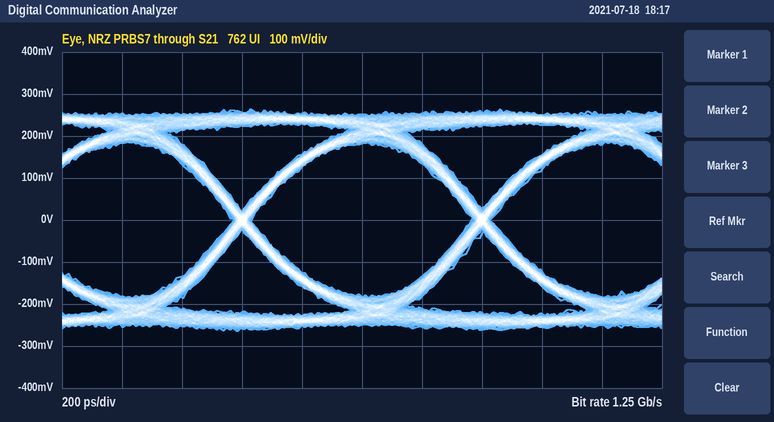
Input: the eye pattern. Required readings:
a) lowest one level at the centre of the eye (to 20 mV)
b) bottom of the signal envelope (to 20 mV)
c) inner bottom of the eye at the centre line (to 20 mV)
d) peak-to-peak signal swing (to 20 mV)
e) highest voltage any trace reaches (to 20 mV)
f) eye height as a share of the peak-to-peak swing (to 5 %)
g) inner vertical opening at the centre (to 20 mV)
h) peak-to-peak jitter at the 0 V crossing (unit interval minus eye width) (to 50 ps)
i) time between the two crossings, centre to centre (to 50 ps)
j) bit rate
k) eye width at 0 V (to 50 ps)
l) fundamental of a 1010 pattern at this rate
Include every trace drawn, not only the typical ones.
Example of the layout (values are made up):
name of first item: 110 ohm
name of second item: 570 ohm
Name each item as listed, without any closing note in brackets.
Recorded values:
lowest one level at the centre of the eye: 180 mV
bottom of the signal envelope: -260 mV
inner bottom of the eye at the centre line: -180 mV
peak-to-peak signal swing: 520 mV
highest voltage any trace reaches: 260 mV
eye height as a share of the peak-to-peak swing: 70 %
inner vertical opening at the centre: 360 mV
peak-to-peak jitter at the 0 V crossing (unit interval minus eye width): 50 ps
time between the two crossings, centre to centre: 800 ps
bit rate: 1.25 Gb/s
eye width at 0 V: 750 ps
fundamental of a 1010 pattern at this rate: 625 MHz
